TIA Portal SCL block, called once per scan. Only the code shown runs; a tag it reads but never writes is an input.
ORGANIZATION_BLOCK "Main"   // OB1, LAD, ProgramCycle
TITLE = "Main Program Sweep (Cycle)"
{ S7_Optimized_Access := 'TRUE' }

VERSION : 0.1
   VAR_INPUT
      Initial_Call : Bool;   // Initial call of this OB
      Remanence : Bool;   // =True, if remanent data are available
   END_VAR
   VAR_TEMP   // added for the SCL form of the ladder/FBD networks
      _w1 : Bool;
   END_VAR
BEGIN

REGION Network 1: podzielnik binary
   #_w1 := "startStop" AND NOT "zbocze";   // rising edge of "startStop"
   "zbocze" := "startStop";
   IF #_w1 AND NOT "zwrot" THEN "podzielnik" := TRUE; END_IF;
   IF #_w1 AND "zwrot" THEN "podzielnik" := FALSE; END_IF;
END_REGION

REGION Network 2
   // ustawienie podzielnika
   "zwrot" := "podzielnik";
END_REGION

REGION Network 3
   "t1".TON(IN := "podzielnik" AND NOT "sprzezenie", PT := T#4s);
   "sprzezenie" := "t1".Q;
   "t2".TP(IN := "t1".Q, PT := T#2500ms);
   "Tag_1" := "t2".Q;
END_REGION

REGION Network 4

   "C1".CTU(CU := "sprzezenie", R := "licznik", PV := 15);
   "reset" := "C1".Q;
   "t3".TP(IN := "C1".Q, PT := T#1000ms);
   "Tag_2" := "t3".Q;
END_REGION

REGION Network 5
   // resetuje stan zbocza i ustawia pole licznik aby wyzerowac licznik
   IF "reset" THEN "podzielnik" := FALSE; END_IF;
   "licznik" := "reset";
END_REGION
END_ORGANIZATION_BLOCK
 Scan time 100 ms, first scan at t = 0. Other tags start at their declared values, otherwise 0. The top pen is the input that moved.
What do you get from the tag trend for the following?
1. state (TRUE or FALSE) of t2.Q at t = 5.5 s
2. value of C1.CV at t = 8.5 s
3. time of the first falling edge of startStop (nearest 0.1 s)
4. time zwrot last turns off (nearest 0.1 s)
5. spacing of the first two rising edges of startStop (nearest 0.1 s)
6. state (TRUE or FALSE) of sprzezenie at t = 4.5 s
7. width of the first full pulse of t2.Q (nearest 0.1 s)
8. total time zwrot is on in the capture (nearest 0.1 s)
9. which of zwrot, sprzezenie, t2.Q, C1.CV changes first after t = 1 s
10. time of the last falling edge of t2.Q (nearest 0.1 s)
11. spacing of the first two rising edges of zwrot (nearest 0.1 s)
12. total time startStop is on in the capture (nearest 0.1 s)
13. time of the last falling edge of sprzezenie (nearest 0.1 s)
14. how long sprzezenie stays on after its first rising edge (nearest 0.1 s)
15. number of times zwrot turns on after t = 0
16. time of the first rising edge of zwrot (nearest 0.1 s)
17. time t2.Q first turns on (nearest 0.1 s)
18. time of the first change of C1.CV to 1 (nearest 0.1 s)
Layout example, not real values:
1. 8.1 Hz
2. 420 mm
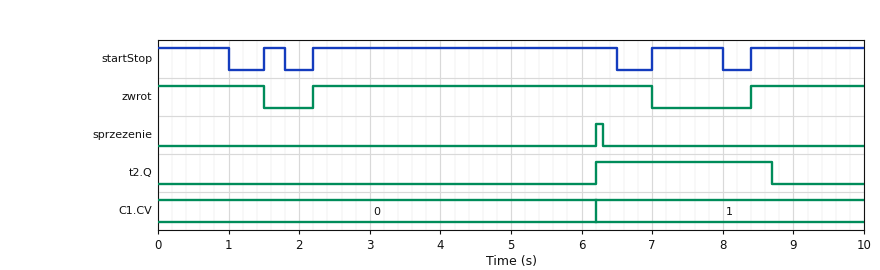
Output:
1. FALSE
2. 1
3. 1.0 s
4. 7.0 s
5. 0.7 s
6. FALSE
7. 2.5 s
8. 7.9 s
9. zwrot
10. 8.7 s
11. 6.2 s
12. 8.2 s
13. 6.3 s
14. 0.1 s
15. 2
16. 2.2 s
17. 6.2 s
18. 6.2 s
